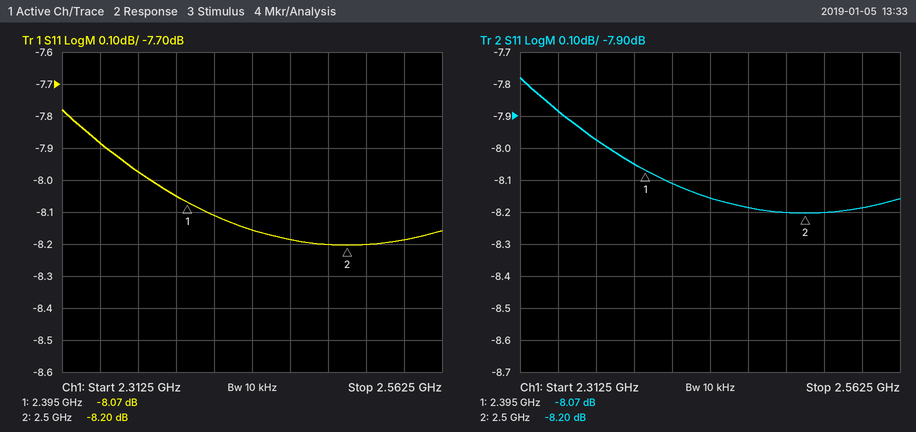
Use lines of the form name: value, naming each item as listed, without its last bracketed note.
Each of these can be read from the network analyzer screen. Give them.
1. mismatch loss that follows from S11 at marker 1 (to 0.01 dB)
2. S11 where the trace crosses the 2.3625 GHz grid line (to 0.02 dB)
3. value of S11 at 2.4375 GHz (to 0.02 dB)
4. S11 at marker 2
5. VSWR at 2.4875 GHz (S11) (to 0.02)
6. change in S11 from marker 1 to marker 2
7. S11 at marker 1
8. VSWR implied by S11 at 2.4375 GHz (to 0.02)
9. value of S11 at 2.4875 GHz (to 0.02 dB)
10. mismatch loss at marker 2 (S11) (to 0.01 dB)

mismatch loss that follows from S11 at marker 1: 0.74 dB
S11 where the trace crosses the 2.3625 GHz grid line: -7.98 dB
value of S11 at 2.4375 GHz: -8.16 dB
S11 at marker 2: -8.20 dB
VSWR at 2.4875 GHz (S11): 2.28
change in S11 from marker 1 to marker 2: -0.13 dB
S11 at marker 1: -8.07 dB
VSWR implied by S11 at 2.4375 GHz: 2.28
value of S11 at 2.4875 GHz: -8.20 dB
mismatch loss at marker 2 (S11): 0.71 dB
